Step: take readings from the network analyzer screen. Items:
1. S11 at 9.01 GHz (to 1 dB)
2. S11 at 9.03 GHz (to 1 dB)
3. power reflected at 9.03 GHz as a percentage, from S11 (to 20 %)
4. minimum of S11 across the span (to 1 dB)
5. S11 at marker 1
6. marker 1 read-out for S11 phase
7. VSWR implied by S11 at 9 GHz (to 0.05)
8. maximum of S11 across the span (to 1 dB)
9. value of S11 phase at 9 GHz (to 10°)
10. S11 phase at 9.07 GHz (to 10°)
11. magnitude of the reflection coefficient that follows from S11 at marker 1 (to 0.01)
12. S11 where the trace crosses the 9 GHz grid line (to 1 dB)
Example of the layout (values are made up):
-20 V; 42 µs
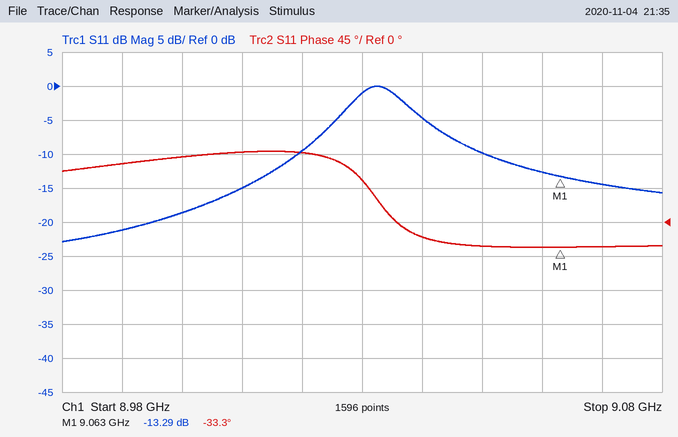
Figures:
-15 dB; -1 dB; 80 %; -23 dB; -13.29 dB; -33.3°; 1.25; 0 dB; 90°; -30°; 0.22; -19 dB
